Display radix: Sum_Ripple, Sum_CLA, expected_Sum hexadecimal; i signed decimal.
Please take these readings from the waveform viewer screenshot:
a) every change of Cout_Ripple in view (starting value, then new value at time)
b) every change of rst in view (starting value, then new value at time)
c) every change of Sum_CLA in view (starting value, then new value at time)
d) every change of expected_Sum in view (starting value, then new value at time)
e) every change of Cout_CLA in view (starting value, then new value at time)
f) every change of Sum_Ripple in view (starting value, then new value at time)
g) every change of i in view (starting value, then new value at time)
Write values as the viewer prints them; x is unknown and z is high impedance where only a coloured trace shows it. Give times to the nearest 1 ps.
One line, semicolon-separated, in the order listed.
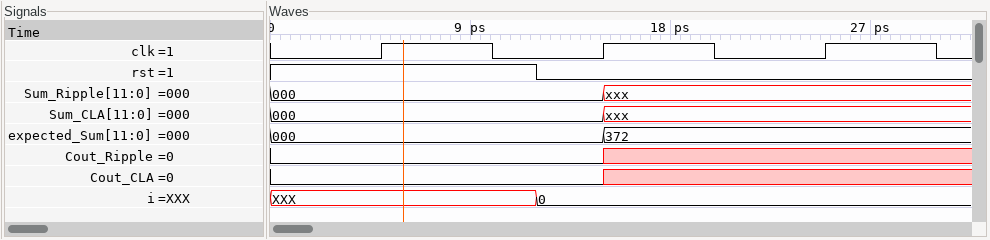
0, x at 15 ps; 1, 0 at 12 ps; 000, xxx at 15 ps; 000, 372 at 15 ps; 0, x at 15 ps; 000, xxx at 15 ps; XXX, 0 at 12 ps
